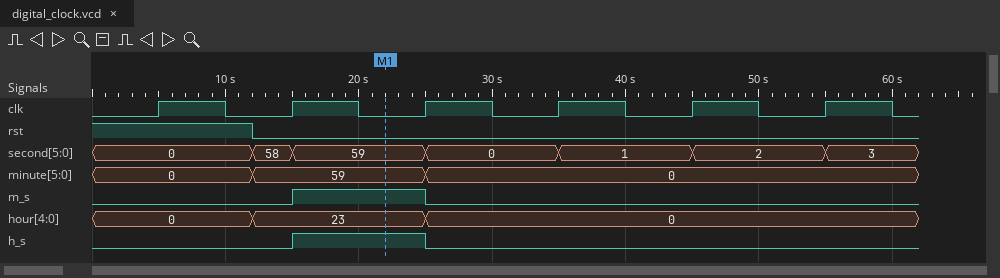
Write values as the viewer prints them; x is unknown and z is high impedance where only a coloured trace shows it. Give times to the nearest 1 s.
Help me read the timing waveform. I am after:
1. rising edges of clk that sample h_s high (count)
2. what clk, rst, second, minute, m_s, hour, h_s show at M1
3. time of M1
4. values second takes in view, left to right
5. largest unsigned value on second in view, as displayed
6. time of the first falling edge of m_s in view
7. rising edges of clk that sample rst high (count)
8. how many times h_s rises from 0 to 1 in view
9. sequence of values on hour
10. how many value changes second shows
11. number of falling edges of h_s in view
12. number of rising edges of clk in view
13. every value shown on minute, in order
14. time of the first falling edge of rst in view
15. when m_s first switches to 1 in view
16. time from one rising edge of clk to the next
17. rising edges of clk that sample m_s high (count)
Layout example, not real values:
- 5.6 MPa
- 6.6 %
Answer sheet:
- 1
- clk=0, rst=0, second=59, minute=59, m_s=1, hour=23, h_s=1
- 22 s
- 0, 58, 59, 0, 1, 2, 3
- 59
- 25 s
- 1
- 1
- 0, 23, 0
- 6
- 1
- 6
- 0, 59, 0
- 12 s
- 15 s
- 10 s
- 1
